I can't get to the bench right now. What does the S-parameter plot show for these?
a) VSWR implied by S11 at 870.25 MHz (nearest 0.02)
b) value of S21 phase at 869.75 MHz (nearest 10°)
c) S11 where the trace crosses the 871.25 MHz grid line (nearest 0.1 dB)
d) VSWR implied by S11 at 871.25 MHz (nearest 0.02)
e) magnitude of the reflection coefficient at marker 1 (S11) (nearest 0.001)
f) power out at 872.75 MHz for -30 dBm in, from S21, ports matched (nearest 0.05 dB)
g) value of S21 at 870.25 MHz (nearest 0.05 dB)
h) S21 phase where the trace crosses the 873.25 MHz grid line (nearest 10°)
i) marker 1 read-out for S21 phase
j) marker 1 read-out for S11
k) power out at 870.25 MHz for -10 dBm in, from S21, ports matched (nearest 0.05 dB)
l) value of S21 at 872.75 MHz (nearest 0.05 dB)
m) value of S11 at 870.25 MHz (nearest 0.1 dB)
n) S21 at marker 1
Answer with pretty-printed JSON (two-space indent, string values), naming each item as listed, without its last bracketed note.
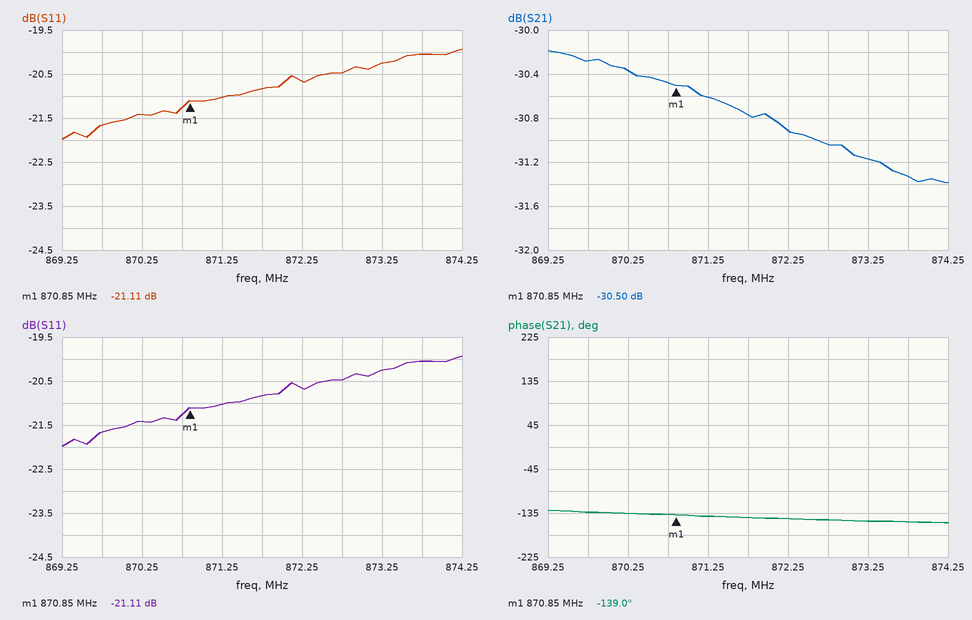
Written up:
{
  "VSWR implied by S11 at 870.25 MHz": "1.18",
  "value of S21 phase at 869.75 MHz": "-130°",
  "S11 where the trace crosses the 871.25 MHz grid line": "-21.0 dB",
  "VSWR implied by S11 at 871.25 MHz": "1.20",
  "magnitude of the reflection coefficient at marker 1 (S11)": "0.088",
  "power out at 872.75 MHz for -30 dBm in, from S21, ports matched": "-61.05 dBm",
  "value of S21 at 870.25 MHz": "-30.35 dB",
  "S21 phase where the trace crosses the 873.25 MHz grid line": "-150°",
  "marker 1 read-out for S21 phase": "-139.0°",
  "marker 1 read-out for S11": "-21.11 dB",
  "power out at 870.25 MHz for -10 dBm in, from S21, ports matched": "-40.35 dBm",
  "value of S21 at 872.75 MHz": "-31.05 dB",
  "value of S11 at 870.25 MHz": "-21.4 dB",
  "S21 at marker 1": "-30.50 dB"
}
